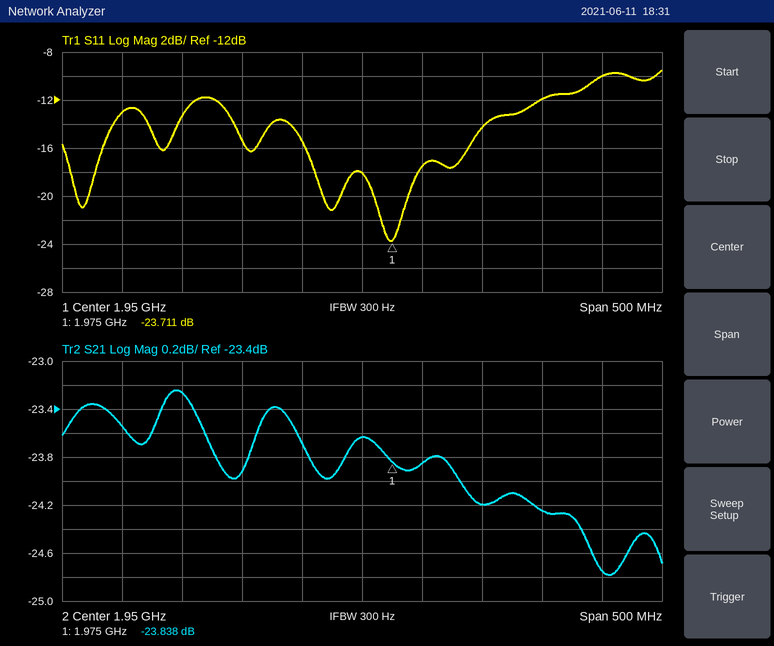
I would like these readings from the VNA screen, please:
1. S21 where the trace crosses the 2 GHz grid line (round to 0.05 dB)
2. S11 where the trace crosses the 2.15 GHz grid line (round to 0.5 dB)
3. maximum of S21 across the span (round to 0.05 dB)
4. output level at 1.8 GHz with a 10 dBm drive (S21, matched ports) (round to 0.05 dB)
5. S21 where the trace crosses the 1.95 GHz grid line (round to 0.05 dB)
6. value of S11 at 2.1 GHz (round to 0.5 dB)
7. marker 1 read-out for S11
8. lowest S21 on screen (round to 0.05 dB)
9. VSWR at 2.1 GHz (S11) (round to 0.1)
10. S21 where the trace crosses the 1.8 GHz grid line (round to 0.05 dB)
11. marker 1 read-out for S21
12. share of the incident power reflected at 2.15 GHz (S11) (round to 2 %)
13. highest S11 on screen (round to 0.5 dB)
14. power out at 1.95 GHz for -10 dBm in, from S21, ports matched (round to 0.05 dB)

-23.85 dB
-10.0 dB
-23.25 dB
-13.25 dBm
-23.65 dB
-12.0 dB
-23.711 dB
-24.80 dB
1.7
-23.25 dB
-23.838 dB
10 %
-9.5 dB
-33.65 dBm
